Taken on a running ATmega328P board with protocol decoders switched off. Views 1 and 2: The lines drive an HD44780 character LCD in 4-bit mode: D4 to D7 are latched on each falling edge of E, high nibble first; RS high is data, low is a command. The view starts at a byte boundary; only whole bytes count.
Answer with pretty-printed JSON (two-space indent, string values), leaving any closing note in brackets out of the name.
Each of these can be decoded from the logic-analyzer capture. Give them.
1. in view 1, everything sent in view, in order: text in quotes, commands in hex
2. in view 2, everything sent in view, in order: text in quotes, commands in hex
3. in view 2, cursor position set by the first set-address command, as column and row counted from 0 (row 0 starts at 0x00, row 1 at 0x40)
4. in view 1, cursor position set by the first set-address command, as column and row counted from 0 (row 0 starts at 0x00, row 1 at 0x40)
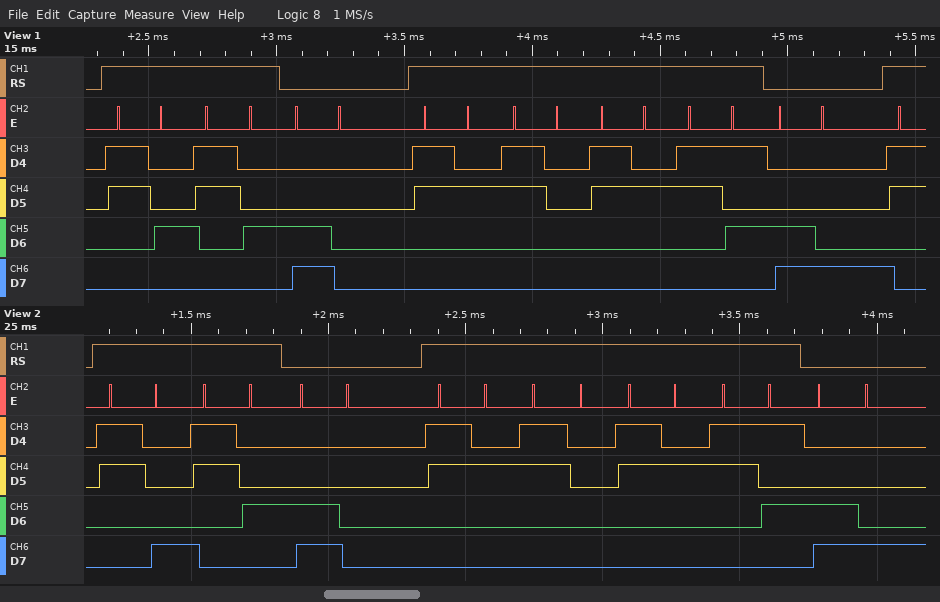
{
  "in view 1, everything sent in view, in order: text in quotes, commands in hex": "\"44\" 0xC0 \"2025\" 0xC8",
  "in view 2, everything sent in view, in order: text in quotes, commands in hex": "\"84\" 0xC0 \"2025\" 0xC8",
  "in view 2, cursor position set by the first set-address command, as column and row counted from 0": "column 0, row 1",
  "in view 1, cursor position set by the first set-address command, as column and row counted from 0": "column 0, row 1"
}
